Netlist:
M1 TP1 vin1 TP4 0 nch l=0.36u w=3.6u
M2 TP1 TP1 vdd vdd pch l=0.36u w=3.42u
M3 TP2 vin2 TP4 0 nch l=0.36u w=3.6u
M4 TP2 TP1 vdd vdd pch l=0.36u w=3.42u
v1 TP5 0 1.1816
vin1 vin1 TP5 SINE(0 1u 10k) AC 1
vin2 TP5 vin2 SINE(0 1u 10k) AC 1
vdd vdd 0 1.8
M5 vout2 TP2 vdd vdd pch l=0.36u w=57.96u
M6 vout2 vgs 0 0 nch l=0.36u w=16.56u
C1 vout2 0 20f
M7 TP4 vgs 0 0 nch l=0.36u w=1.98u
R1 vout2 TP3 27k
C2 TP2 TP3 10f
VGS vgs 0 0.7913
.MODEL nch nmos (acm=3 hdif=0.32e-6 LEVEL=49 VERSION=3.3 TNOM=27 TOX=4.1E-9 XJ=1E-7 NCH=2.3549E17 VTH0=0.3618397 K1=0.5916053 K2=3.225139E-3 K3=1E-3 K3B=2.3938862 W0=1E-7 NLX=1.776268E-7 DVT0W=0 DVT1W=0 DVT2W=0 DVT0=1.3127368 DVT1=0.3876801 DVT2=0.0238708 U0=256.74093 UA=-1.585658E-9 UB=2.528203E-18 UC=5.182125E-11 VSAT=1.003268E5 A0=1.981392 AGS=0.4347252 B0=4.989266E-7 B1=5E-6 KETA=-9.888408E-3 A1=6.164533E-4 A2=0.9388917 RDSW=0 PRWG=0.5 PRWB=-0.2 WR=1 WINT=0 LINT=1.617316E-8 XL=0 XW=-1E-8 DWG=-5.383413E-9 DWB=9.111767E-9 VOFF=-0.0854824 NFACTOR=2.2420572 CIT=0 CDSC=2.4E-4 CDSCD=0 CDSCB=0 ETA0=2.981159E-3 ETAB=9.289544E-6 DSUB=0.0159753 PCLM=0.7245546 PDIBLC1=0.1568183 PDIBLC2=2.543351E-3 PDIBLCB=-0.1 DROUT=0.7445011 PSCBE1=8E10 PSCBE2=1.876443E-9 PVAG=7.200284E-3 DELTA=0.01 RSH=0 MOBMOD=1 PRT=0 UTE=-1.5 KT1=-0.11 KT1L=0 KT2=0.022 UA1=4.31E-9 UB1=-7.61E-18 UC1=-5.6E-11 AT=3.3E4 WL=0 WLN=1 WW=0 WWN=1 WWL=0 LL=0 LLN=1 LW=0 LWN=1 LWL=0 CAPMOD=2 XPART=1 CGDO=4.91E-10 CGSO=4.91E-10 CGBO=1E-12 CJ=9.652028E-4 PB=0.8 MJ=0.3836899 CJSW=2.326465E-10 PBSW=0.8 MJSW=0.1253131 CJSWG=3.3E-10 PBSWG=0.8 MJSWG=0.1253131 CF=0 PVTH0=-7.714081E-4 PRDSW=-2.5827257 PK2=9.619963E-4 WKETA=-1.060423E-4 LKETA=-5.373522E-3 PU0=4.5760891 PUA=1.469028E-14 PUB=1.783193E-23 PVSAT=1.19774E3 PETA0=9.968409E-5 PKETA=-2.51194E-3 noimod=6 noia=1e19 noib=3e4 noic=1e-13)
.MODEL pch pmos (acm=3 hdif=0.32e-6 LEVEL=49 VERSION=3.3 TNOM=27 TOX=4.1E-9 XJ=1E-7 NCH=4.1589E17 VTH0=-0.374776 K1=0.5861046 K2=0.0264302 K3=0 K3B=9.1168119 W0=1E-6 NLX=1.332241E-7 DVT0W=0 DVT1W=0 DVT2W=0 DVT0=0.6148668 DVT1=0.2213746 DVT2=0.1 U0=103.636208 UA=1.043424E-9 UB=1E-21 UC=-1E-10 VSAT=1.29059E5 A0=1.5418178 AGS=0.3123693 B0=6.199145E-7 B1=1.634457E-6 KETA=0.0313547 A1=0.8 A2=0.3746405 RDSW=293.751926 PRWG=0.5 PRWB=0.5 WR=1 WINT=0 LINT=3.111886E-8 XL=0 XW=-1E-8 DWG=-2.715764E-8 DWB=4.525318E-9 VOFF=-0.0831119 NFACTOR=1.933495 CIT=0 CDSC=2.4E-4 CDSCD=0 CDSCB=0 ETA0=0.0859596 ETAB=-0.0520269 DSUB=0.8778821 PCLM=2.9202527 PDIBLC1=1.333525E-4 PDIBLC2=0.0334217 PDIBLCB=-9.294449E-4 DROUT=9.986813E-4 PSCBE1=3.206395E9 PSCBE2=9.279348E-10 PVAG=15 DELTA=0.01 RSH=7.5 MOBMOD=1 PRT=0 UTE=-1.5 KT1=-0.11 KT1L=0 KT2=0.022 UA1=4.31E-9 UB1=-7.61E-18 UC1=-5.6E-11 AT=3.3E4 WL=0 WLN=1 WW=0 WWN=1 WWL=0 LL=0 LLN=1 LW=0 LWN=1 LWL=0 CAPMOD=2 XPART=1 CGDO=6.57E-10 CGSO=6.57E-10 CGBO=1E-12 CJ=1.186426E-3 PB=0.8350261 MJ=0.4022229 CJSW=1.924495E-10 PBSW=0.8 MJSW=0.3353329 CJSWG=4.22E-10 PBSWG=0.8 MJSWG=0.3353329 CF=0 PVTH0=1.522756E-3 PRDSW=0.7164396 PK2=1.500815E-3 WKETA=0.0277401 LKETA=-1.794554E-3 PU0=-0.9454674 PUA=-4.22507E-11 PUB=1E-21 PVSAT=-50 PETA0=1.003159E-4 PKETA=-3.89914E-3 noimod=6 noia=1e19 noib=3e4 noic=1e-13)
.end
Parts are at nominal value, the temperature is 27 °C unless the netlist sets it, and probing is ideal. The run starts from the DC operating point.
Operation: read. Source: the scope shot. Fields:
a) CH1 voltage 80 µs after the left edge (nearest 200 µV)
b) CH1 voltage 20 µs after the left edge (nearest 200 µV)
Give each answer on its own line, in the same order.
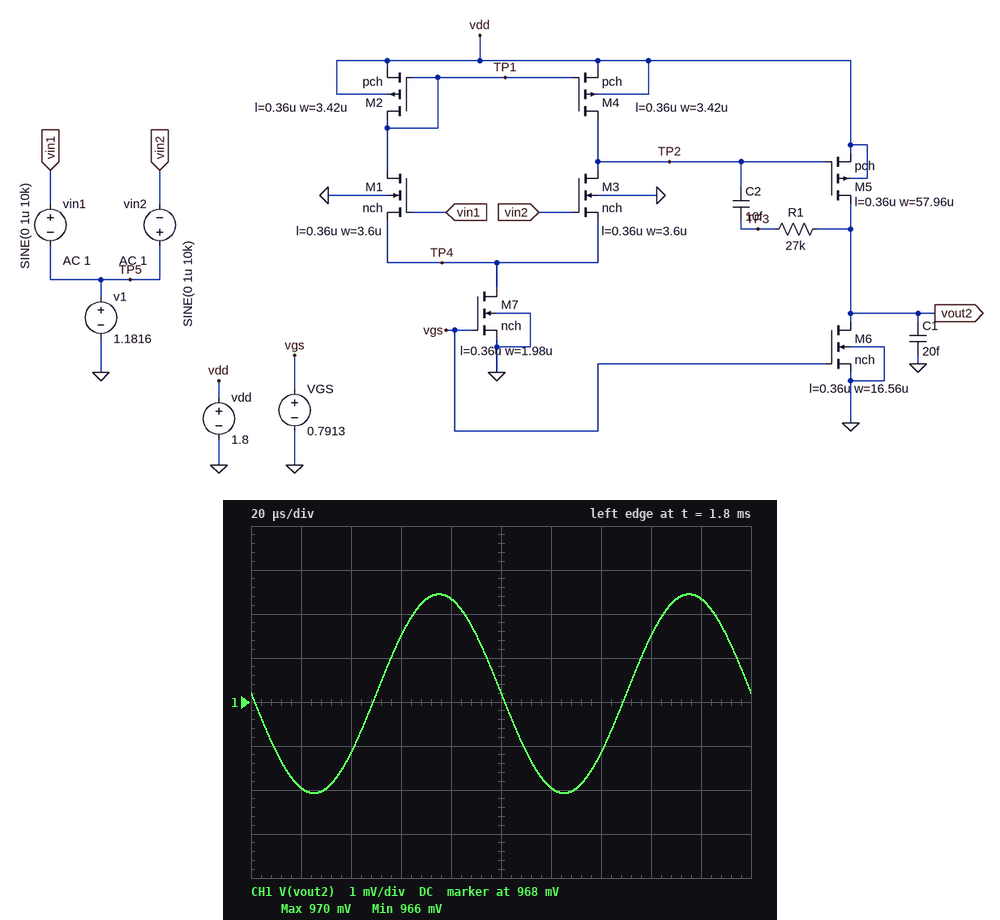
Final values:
970.4 mV
966.0 mV
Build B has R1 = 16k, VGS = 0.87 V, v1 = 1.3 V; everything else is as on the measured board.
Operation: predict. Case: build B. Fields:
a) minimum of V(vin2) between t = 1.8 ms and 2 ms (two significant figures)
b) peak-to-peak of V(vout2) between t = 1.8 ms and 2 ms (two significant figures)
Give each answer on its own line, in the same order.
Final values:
1.3 V
3.3 mV
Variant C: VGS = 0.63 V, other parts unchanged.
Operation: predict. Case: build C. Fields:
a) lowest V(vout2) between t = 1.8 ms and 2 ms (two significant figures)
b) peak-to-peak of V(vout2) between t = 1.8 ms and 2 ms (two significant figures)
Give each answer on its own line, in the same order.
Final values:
1.0 V
6.6 mV
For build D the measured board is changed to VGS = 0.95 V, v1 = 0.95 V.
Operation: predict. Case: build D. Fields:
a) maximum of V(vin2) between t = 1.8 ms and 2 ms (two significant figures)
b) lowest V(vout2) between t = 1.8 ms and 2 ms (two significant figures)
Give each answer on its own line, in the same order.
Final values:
950 mV
280 mV
